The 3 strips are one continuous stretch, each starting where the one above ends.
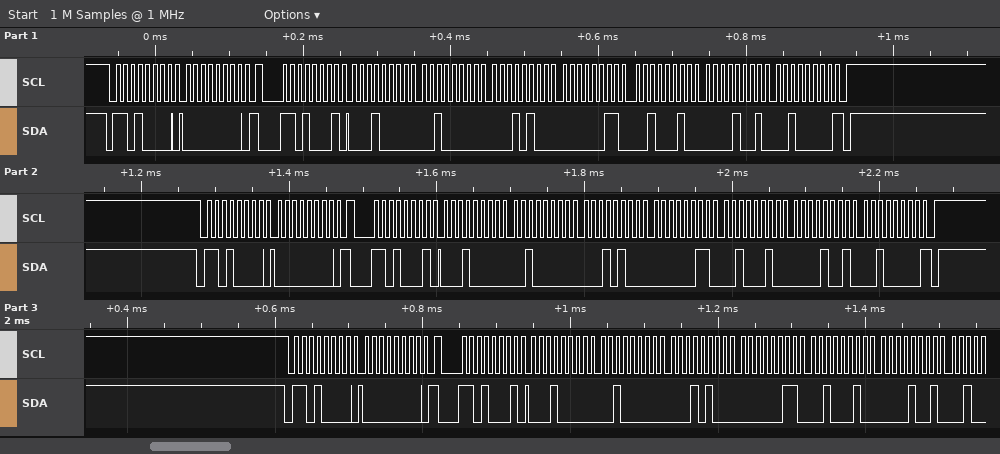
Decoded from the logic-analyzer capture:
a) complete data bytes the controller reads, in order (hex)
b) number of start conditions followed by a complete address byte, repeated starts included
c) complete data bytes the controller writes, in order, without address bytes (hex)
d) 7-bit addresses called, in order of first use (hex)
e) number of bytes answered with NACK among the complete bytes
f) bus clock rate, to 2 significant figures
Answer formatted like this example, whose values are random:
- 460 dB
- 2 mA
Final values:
- 10 20 14 03 22 09 20 10 20 14 03 22 09 20 10 20 14 03 22 09
- 6
- 00 00 00
- 0x68
- 2
- 100 kHz
